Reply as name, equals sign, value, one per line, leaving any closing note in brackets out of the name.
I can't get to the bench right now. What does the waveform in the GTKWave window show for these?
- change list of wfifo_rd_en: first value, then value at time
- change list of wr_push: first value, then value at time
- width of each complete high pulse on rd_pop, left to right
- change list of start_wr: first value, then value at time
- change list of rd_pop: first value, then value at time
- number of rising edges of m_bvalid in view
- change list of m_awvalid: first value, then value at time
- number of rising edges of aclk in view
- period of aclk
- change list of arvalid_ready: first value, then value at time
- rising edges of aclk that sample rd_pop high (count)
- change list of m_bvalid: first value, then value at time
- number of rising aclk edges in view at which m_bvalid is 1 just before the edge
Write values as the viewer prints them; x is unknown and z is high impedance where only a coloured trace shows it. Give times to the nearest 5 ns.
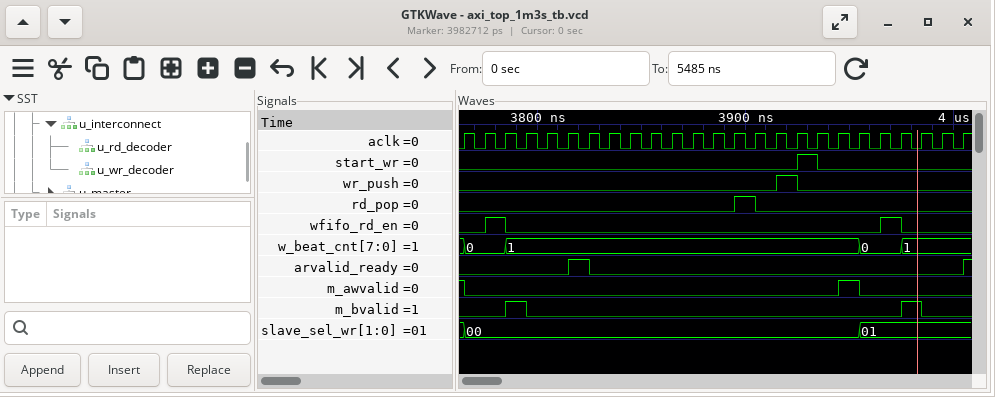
change list of wfifo_rd_en: first value, then value at time = 0, 1 at 3775 ns, 0 at 3785 ns, 1 at 3965 ns, 0 at 3975 ns
change list of wr_push: first value, then value at time = 0, 1 at 3915 ns, 0 at 3925 ns
width of each complete high pulse on rd_pop, left to right = 10 ns
change list of start_wr: first value, then value at time = 0, 1 at 3925 ns, 0 at 3935 ns
change list of rd_pop: first value, then value at time = 0, 1 at 3895 ns, 0 at 3905 ns
number of rising edges of m_bvalid in view = 2
change list of m_awvalid: first value, then value at time = 1, 0 at 3765 ns, 1 at 3945 ns, 0 at 3955 ns
number of rising edges of aclk in view = 25
period of aclk = 10 ns
change list of arvalid_ready: first value, then value at time = 0, 1 at 3815 ns, 0 at 3825 ns, 1 at 4005 ns
rising edges of aclk that sample rd_pop high = 1
change list of m_bvalid: first value, then value at time = 0, 1 at 3785 ns, 0 at 3795 ns, 1 at 3975 ns, 0 at 3985 ns
number of rising aclk edges in view at which m_bvalid is 1 just before the edge = 2
